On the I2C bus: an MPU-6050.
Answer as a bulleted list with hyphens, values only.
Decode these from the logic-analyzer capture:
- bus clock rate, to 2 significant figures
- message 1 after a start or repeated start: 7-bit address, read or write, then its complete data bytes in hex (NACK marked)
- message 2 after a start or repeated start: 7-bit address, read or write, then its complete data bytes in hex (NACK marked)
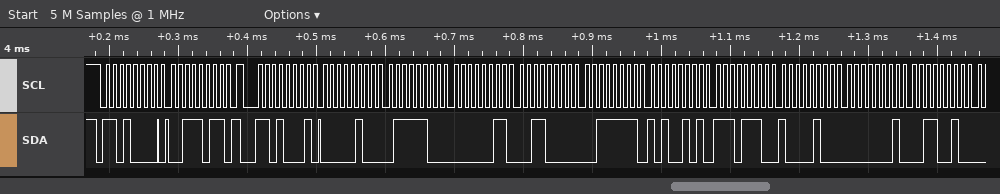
- 100 kHz
- 0x68 write: 3B
- 0x68 read: 04 7C 03 30 3F A5 EE 84 01 32
